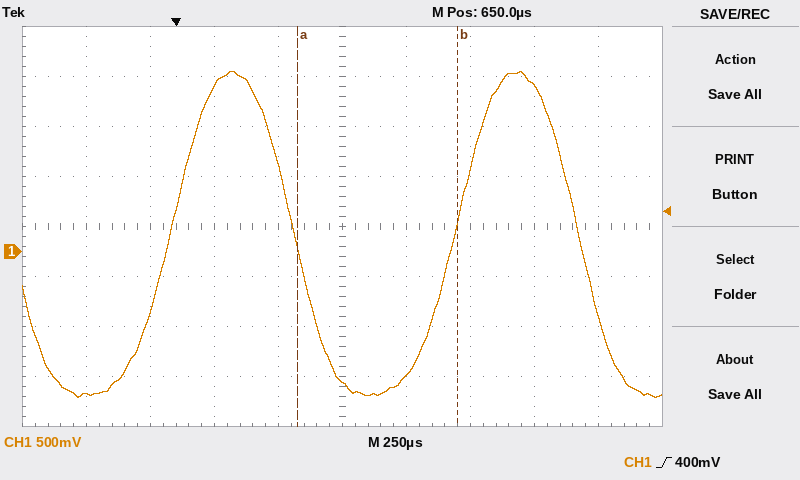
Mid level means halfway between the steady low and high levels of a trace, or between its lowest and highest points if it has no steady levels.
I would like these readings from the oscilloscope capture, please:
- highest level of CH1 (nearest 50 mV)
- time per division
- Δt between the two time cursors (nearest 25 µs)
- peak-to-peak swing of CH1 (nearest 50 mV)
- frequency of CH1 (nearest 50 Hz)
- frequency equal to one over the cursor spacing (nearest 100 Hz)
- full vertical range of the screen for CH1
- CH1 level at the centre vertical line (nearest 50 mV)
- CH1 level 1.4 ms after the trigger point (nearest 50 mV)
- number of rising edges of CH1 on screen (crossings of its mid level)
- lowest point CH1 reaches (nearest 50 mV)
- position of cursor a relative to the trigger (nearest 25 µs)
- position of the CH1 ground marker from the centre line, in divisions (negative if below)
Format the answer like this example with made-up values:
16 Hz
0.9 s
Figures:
1.80 V
250 µs
625 µs
3.25 V
900 Hz
1.6 kHz
4 V
-1.30 V
1.65 V
2
-1.45 V
+475 µs
-0.5 div
